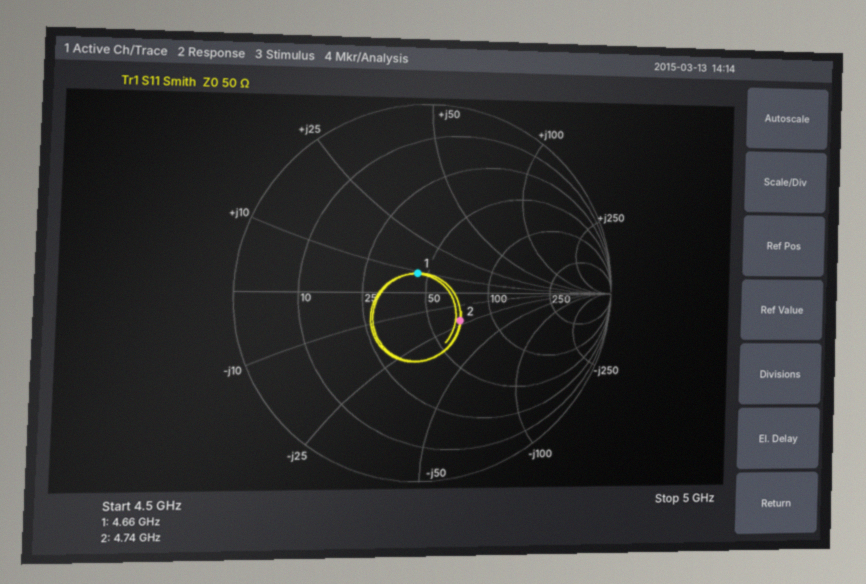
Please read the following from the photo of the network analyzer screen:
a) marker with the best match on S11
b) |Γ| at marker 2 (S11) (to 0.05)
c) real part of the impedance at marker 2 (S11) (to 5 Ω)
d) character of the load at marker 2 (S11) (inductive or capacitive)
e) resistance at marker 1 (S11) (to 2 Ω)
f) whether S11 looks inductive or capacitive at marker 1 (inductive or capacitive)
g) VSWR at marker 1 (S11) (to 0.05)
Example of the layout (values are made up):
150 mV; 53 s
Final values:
marker 1; 0.25; 70 Ω; capacitive; 44 Ω; inductive; 1.25
